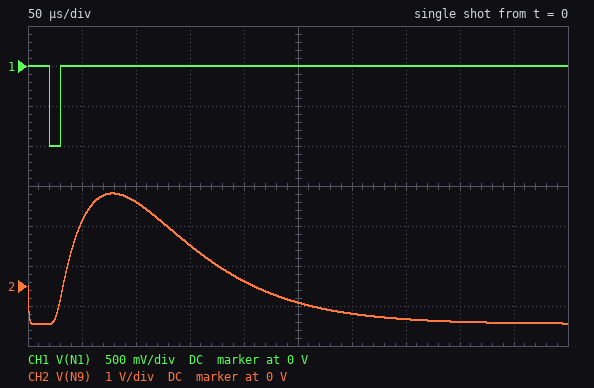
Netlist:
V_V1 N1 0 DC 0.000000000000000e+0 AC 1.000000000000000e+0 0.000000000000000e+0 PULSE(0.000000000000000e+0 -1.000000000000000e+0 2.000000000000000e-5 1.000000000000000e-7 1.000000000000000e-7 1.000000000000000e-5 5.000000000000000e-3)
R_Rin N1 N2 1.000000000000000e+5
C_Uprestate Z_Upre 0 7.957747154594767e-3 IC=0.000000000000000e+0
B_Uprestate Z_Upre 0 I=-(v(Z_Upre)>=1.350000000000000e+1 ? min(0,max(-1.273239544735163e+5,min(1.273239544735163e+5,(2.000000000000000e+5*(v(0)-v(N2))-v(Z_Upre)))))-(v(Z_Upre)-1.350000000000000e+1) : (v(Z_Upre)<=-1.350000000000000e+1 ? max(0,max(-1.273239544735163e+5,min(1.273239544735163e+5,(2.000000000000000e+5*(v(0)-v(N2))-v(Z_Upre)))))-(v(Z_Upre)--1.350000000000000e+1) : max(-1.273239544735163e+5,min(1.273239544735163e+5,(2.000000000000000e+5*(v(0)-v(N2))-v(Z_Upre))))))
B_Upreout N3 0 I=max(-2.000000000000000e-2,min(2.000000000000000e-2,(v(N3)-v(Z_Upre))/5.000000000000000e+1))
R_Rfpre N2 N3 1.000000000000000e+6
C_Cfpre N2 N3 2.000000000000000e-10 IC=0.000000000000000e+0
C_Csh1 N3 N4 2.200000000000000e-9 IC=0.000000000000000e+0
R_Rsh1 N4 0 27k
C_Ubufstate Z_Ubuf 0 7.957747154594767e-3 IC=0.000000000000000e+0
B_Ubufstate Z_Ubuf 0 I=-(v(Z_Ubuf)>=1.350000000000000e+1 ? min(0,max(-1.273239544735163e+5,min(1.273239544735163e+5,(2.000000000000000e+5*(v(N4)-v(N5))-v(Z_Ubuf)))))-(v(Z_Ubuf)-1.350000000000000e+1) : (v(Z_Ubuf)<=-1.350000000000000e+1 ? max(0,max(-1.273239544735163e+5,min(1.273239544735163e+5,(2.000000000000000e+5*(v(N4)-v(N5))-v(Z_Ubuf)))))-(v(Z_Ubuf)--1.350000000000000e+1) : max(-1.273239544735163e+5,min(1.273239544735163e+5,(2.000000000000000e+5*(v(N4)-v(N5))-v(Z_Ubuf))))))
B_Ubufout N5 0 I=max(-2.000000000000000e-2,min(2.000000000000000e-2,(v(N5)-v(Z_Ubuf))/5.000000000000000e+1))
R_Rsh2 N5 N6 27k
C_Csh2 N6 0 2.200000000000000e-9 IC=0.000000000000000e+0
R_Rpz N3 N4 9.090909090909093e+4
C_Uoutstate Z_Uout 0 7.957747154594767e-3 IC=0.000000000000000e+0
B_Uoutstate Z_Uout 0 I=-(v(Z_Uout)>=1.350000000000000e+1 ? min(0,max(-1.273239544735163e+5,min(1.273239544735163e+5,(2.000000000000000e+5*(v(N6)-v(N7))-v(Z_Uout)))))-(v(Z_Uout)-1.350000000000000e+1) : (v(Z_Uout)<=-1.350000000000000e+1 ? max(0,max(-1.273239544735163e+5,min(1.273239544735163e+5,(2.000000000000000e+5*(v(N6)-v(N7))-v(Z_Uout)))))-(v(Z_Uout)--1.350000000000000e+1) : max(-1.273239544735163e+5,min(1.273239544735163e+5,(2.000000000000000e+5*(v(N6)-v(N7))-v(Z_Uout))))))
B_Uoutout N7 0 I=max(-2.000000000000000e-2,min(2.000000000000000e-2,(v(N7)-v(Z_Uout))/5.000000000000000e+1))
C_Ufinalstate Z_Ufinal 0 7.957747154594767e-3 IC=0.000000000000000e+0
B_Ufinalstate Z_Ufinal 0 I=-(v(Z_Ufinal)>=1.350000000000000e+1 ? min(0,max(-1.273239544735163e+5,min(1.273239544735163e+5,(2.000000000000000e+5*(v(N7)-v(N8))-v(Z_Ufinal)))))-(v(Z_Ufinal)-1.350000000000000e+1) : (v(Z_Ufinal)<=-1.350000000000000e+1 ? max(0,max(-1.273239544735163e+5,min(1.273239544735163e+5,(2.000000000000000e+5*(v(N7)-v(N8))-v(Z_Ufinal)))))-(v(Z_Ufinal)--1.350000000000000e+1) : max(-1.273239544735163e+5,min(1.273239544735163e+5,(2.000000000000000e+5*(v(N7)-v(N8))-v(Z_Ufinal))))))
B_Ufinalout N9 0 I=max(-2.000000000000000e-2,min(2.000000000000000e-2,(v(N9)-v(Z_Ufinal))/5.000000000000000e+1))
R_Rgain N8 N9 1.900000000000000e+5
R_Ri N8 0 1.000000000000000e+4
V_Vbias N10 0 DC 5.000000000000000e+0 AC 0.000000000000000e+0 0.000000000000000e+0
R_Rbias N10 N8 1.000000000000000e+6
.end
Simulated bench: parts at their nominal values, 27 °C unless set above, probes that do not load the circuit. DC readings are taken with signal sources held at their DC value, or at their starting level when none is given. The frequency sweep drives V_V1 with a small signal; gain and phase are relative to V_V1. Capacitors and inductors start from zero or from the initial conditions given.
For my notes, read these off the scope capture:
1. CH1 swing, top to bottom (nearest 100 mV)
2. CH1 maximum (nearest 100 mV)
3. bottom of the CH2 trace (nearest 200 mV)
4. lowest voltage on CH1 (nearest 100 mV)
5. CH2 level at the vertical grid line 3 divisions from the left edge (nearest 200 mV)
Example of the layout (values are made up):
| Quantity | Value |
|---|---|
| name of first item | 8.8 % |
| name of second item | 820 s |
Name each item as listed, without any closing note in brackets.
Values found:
| Quantity | Value |
|---|---|
| CH1 swing, top to bottom | 1.0 V |
| CH1 maximum | 0 V |
| bottom of the CH2 trace | -1.0 V |
| lowest voltage on CH1 | -1.0 V |
| CH2 level at the vertical grid line 3 divisions from the left edge | 1.0 V |
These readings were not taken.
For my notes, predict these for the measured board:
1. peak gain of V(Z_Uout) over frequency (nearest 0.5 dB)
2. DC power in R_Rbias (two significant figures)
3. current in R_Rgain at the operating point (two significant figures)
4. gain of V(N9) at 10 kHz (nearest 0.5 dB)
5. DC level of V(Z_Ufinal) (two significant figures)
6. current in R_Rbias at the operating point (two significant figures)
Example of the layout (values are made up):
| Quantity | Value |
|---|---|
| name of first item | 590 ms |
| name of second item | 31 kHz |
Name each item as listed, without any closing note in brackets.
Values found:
| Quantity | Value |
|---|---|
| peak gain of V(Z_Uout) over frequency | 7.0 dB |
| DC power in R_Rbias | 25 µW |
| current in R_Rgain at the operating point | 5.0 µA |
| gain of V(N9) at 10 kHz | 12.0 dB |
| DC level of V(Z_Ufinal) | -950 mV |
| current in R_Rbias at the operating point | 5.0 µA |
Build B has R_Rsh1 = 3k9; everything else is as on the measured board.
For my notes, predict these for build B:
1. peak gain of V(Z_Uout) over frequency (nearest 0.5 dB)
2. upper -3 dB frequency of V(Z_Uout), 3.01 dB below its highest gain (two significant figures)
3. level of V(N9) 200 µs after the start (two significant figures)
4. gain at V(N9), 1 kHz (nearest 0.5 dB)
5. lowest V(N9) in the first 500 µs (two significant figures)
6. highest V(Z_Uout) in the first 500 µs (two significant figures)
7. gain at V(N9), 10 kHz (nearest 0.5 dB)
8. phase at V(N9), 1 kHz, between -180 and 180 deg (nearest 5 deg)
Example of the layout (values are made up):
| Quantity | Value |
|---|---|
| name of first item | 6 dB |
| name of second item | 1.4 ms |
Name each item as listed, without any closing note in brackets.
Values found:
| Quantity | Value |
|---|---|
| peak gain of V(Z_Uout) over frequency | -7.5 dB |
| upper -3 dB frequency of V(Z_Uout), 3.01 dB below its highest gain | 2.6 kHz |
| level of V(N9) 200 µs after the start | -860 mV |
| gain at V(N9), 1 kHz | 18.0 dB |
| lowest V(N9) in the first 500 µs | -950 mV |
| highest V(Z_Uout) in the first 500 µs | 50 mV |
| gain at V(N9), 10 kHz | 5.5 dB |
| phase at V(N9), 1 kHz, between -180 and 180 deg | 155 deg |
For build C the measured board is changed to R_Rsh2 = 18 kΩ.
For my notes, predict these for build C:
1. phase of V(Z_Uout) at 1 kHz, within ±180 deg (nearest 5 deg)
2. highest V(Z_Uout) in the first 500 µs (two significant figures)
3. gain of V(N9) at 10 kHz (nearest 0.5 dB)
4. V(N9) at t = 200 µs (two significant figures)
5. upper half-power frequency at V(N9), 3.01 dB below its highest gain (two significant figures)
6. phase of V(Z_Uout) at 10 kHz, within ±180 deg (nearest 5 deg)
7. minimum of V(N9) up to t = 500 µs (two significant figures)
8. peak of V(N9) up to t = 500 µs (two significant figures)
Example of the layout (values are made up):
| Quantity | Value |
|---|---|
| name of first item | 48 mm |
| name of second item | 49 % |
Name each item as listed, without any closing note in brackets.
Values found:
| Quantity | Value |
|---|---|
| phase of V(Z_Uout) at 1 kHz, within ±180 deg | 150 deg |
| highest V(Z_Uout) in the first 500 µs | 200 mV |
| gain of V(N9) at 10 kHz | 15.0 dB |
| V(N9) at t = 200 µs | -190 mV |
| upper half-power frequency at V(N9), 3.01 dB below its highest gain | 2.4 kHz |
| phase of V(Z_Uout) at 10 kHz, within ±180 deg | 40 deg |
| minimum of V(N9) up to t = 500 µs | -950 mV |
| peak of V(N9) up to t = 500 µs | 3.1 V |
